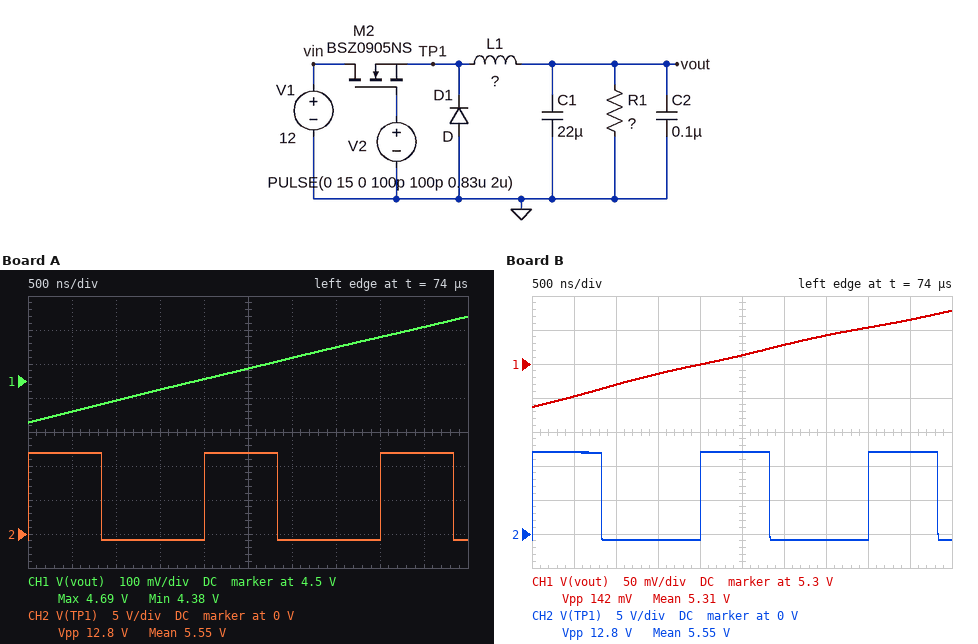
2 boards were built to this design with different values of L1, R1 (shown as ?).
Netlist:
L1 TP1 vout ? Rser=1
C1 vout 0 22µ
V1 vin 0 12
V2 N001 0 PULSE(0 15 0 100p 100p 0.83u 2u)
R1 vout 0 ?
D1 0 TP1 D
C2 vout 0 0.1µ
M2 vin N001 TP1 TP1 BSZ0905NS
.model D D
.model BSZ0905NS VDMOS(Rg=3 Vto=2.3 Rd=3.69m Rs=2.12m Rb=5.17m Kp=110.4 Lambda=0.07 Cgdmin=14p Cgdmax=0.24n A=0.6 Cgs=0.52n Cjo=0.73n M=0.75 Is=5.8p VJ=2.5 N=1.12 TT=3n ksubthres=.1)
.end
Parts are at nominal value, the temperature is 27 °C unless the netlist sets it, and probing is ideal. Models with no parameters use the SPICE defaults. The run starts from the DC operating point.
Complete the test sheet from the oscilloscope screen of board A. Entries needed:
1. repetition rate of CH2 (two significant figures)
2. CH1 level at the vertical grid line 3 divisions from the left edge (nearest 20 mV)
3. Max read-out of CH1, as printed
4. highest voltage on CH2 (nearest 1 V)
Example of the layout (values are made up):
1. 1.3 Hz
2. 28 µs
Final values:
1. 500 kHz
2. 4.48 V
3. 4.69 V
4. 12 V
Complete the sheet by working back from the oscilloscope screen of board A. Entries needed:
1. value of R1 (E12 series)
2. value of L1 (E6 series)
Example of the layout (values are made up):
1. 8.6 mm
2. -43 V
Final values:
1. 68 Ω
2. 68 µH
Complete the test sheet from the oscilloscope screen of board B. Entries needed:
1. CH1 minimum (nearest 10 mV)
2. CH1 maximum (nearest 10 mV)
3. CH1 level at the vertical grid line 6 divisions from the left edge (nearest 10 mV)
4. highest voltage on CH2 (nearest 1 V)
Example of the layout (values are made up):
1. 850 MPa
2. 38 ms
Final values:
1. 5.24 V
2. 5.38 V
3. 5.33 V
4. 12 V
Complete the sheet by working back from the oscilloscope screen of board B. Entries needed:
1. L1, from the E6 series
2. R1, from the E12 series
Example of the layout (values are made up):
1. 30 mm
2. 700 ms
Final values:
1. 33 µH
2. 150 Ω
